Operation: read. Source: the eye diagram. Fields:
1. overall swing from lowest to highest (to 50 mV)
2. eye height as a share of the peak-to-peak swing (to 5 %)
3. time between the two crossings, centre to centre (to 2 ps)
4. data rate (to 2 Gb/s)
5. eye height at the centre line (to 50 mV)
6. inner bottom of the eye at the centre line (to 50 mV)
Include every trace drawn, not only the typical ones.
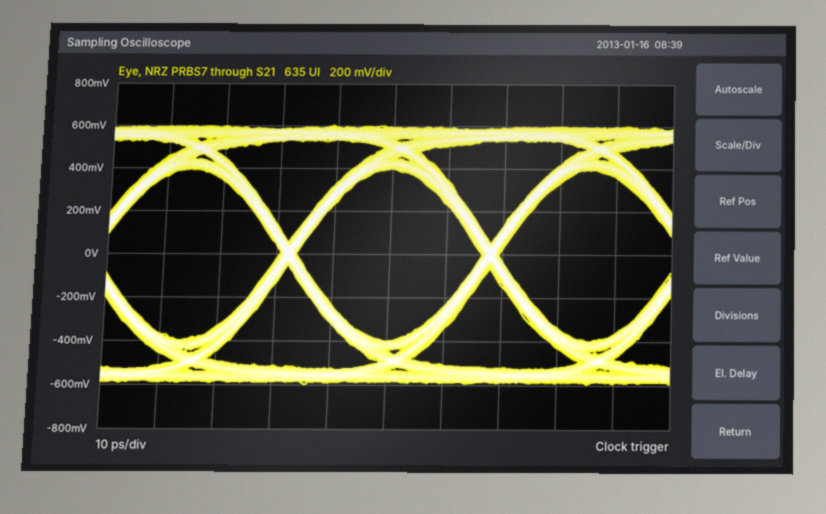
1.20 V
65 %
36 ps
28 Gb/s
800 mV
-400 mV
